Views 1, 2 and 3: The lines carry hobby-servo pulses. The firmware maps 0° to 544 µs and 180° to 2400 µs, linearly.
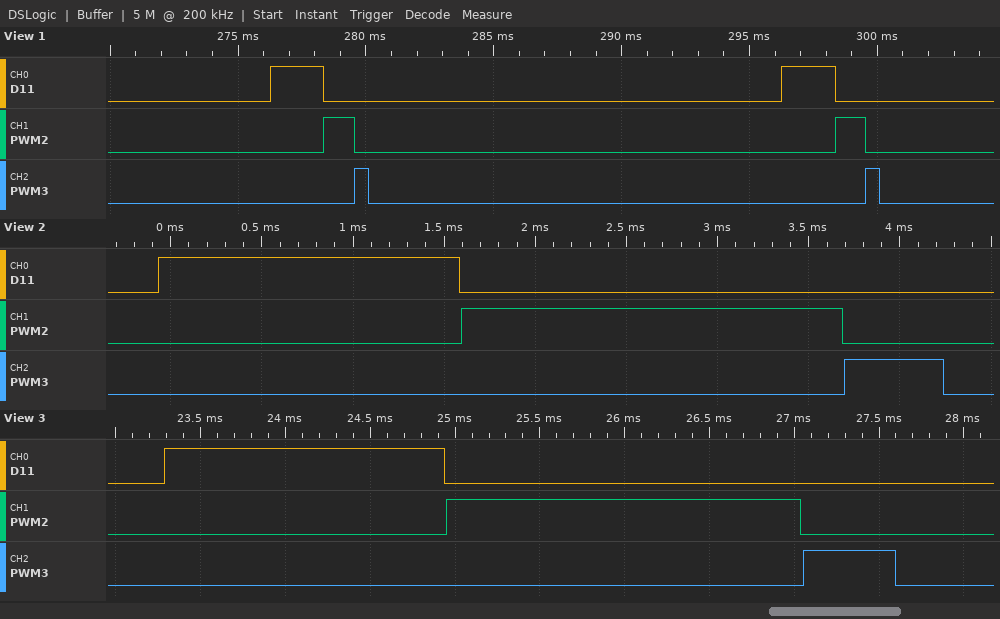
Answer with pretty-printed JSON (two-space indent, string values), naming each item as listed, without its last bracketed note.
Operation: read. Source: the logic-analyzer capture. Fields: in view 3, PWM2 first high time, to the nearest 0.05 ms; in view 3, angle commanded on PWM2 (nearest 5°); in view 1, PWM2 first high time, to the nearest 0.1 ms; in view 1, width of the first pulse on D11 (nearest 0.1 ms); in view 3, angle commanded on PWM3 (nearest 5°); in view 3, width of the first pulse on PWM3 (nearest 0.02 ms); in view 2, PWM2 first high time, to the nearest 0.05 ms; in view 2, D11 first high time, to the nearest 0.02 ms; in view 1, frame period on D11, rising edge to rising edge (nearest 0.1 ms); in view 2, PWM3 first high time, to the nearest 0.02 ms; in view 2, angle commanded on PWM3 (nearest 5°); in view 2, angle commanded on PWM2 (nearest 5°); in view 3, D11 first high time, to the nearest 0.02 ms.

{
  "in view 3, PWM2 first high time, to the nearest 0.05 ms": "2.10 ms",
  "in view 3, angle commanded on PWM2": "150°",
  "in view 1, PWM2 first high time, to the nearest 0.1 ms": "1.2 ms",
  "in view 1, width of the first pulse on D11": "2.1 ms",
  "in view 3, angle commanded on PWM3": "0°",
  "in view 3, width of the first pulse on PWM3": "0.54 ms",
  "in view 2, PWM2 first high time, to the nearest 0.05 ms": "2.10 ms",
  "in view 2, D11 first high time, to the nearest 0.02 ms": "1.66 ms",
  "in view 1, frame period on D11, rising edge to rising edge": "20.0 ms",
  "in view 2, PWM3 first high time, to the nearest 0.02 ms": "0.54 ms",
  "in view 2, angle commanded on PWM3": "0°",
  "in view 2, angle commanded on PWM2": "150°",
  "in view 3, D11 first high time, to the nearest 0.02 ms": "1.66 ms"
}
